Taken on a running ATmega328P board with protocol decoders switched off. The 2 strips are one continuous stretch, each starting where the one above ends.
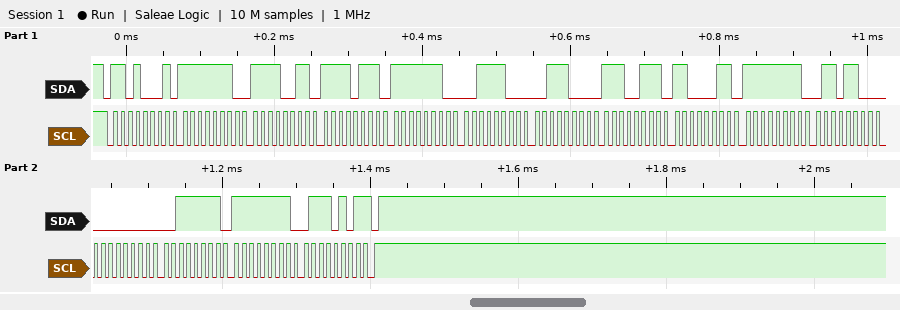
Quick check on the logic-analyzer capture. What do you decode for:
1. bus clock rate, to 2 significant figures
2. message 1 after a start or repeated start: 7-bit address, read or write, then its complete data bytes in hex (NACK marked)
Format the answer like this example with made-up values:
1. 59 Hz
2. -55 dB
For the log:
1. 100 kHz
2. 0x68 read: FE F3 F7 FE 3C 38 E7 C3 FF 6C 00 3F FF 75 NACK
